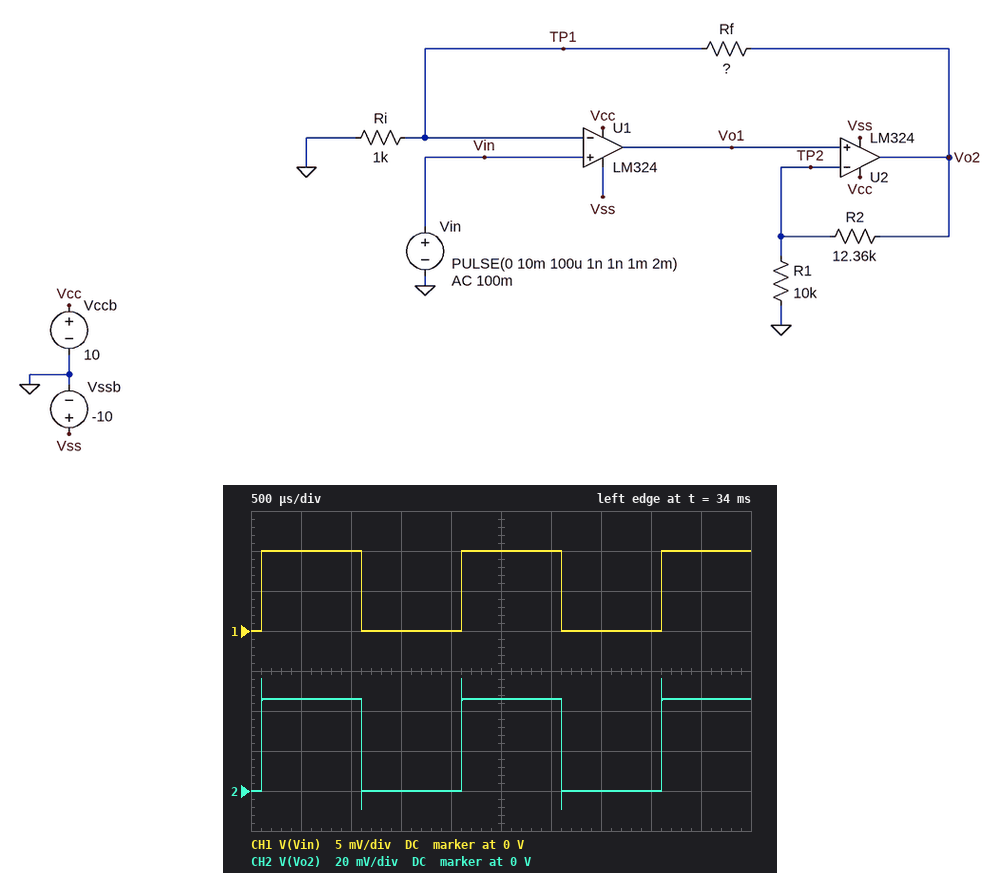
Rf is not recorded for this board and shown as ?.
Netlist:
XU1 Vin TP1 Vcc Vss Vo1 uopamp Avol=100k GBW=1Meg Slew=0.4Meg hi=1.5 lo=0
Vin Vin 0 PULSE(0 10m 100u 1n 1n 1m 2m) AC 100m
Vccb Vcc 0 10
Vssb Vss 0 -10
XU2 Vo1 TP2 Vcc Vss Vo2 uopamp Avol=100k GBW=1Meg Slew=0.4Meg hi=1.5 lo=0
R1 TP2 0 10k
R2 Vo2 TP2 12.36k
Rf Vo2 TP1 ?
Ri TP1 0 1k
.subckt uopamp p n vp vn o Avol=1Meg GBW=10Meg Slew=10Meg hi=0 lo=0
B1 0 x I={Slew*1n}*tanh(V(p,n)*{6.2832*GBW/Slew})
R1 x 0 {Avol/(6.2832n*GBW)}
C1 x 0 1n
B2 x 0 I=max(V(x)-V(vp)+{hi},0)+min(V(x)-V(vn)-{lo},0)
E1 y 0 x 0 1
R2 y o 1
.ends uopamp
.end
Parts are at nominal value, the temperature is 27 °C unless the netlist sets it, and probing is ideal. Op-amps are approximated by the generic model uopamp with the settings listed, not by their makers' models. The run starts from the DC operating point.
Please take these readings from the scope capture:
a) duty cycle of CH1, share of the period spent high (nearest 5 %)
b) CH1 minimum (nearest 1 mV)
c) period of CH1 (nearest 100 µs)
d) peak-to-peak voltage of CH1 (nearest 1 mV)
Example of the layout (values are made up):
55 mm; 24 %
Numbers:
50 %; 0 V; 2.0 ms; 10 mV
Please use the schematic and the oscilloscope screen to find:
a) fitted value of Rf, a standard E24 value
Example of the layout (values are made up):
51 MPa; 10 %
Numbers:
3.6 kΩ
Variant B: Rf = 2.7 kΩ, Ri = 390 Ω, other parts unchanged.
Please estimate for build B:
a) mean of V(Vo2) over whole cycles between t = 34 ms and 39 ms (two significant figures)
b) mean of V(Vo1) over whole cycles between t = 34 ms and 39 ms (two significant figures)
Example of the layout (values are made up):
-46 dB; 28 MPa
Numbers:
40 mV; 18 mV
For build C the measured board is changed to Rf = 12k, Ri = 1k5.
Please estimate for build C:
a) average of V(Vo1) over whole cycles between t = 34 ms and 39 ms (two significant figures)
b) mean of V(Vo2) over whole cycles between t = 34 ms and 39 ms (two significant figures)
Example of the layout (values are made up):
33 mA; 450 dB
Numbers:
20 mV; 45 mV
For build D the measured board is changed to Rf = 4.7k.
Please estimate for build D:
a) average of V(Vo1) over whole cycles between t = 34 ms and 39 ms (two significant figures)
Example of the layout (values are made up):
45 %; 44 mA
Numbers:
13 mV
